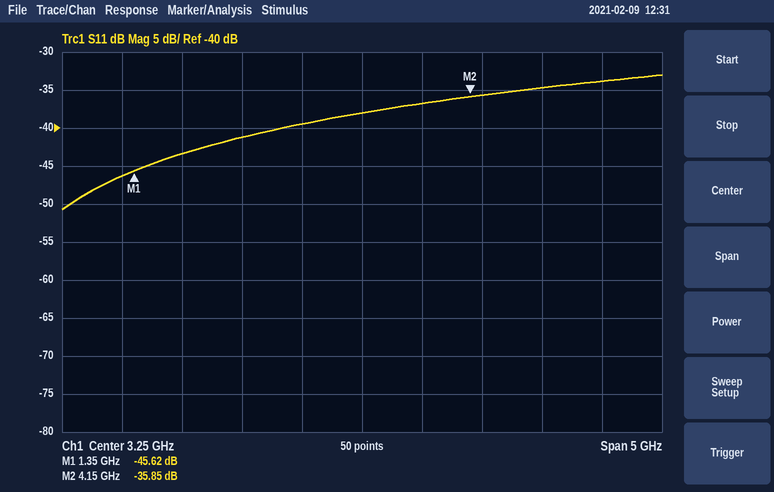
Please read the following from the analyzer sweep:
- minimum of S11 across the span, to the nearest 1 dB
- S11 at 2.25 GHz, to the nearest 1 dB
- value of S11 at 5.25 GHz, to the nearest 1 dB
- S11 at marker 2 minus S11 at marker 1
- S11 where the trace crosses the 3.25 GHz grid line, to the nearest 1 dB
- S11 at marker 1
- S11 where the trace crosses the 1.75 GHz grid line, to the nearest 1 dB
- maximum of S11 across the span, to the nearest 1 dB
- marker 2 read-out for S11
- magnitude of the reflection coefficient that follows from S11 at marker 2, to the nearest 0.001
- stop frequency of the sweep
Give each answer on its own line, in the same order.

-51 dB
-41 dB
-34 dB
9.77 dB
-38 dB
-45.62 dB
-43 dB
-33 dB
-35.85 dB
0.016
5.75 GHz
